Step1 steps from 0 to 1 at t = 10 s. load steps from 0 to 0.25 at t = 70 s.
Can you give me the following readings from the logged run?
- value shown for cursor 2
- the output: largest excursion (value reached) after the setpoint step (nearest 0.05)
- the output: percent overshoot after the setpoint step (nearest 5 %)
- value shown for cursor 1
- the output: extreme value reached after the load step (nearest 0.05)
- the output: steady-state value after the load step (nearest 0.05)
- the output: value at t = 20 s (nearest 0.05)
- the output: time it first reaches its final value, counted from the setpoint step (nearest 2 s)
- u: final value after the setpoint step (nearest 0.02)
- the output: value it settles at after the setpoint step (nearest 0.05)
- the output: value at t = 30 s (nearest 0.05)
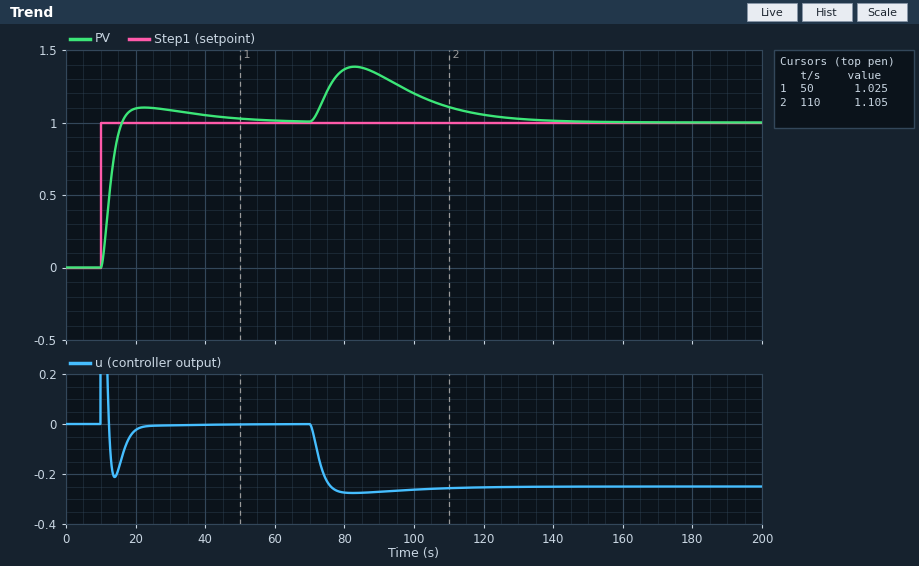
1.105
1.10
10 %
1.025
1.40
1.00
1.10
6 s
0.00
1.00
1.10
